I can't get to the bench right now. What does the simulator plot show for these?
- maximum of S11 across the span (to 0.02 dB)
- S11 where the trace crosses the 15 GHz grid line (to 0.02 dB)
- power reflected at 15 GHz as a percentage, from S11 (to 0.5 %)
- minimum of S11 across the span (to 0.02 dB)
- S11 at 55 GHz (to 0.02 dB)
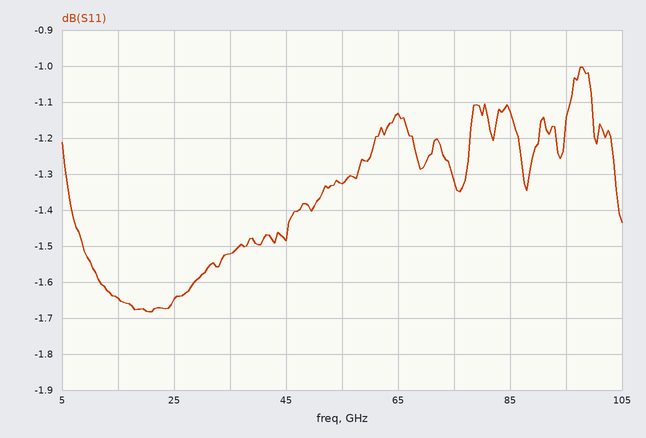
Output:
-1.00 dB
-1.64 dB
68.5 %
-1.68 dB
-1.32 dB
